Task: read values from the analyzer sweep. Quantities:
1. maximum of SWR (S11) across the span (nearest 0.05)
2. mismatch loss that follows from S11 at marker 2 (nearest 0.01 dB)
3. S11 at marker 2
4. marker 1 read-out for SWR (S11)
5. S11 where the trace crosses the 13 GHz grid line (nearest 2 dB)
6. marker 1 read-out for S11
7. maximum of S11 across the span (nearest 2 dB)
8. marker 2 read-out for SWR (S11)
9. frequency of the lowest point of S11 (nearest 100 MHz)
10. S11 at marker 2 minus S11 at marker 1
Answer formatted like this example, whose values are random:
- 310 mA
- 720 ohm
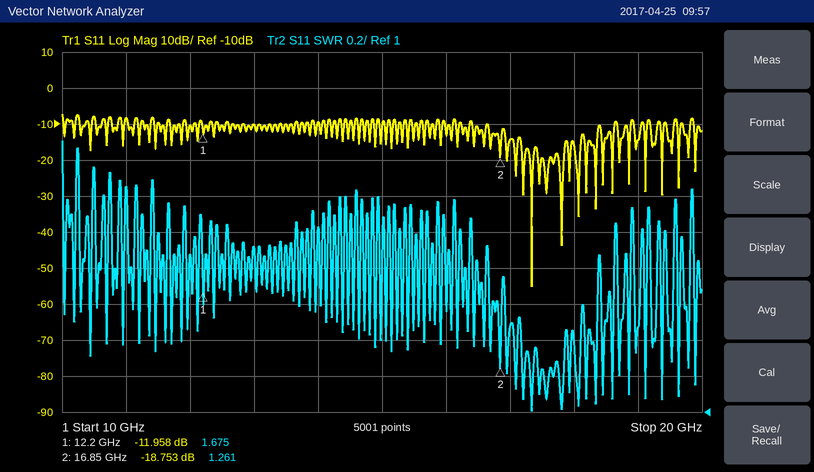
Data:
- 2.50
- 0.06 dB
- -18.753 dB
- 1.675
- -10 dB
- -11.958 dB
- -8 dB
- 1.261
- 17.3 GHz
- -6.795 dB
